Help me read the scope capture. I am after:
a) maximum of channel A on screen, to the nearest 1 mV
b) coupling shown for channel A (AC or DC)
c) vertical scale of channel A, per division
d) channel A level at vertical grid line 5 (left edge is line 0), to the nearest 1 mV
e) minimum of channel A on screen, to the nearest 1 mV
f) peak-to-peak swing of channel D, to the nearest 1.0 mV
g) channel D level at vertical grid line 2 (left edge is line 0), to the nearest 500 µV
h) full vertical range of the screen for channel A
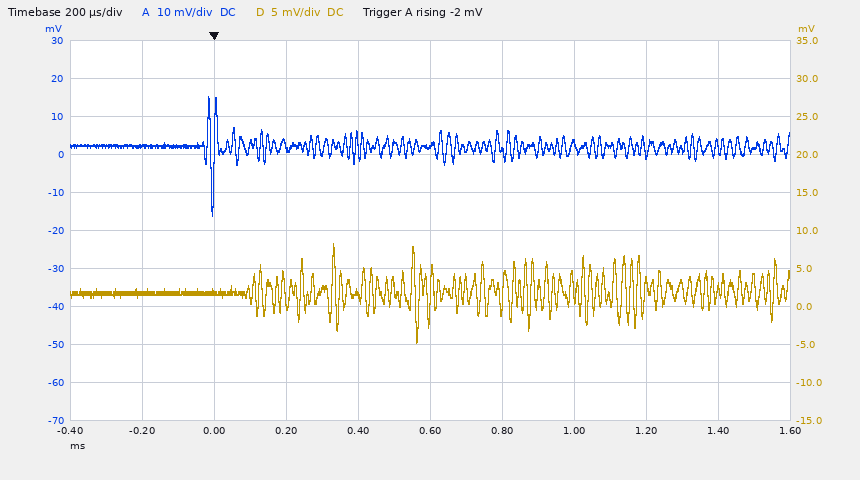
15 mV
DC
10 mV
2 mV
-16 mV
13.0 mV
2.0 mV
100 mV
